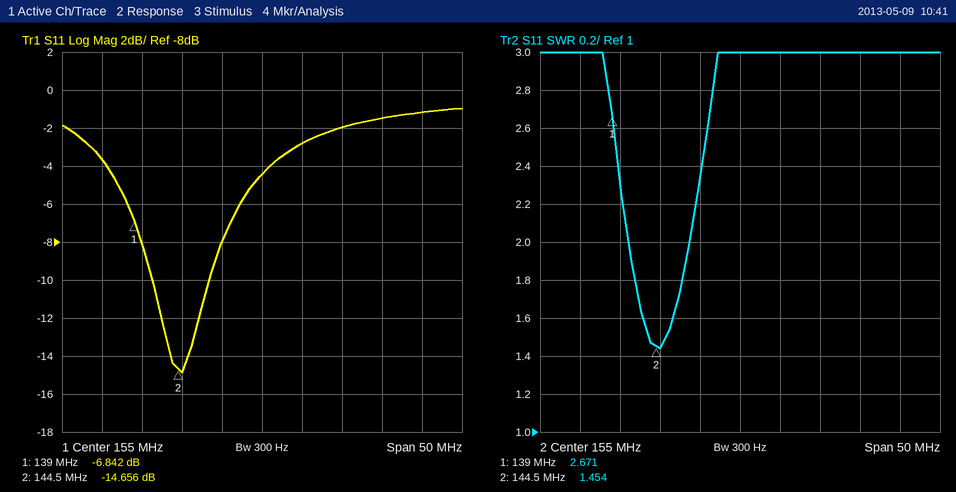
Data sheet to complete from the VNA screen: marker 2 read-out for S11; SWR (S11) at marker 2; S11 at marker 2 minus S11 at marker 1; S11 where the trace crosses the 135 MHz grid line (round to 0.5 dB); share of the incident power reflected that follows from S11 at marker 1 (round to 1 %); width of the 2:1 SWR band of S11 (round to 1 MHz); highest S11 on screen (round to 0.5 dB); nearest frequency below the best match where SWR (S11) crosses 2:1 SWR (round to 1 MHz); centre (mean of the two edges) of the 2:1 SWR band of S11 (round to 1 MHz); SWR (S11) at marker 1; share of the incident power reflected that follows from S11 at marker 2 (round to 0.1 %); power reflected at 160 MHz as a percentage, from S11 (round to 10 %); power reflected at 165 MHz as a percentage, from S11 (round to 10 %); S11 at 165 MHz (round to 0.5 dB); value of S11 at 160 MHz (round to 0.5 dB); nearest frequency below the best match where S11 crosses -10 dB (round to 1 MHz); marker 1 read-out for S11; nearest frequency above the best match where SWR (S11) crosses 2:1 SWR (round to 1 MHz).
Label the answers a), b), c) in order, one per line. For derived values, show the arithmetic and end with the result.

a) -14.656 dB
b) 1.454
c) -14.656 − (-6.842) = -7.814 dB
d) -3.5 dB
e) 10^(-6.842/10) ≈ 21 %
f) 149 MHz − 141 MHz = 8 MHz
g) -1.0 dB
h) 141 MHz
i) 145 MHz
j) 2.671
k) 10^(-14.656/10) ≈ 3.4 %
l) 10^(-3/10) ≈ 50 %
m) 10^(-2/10) ≈ 63.1 %, so 60 % to the nearest 10 %
n) -2.0 dB
o) -3.0 dB
p) 141 MHz
q) -6.842 dB
r) 149 MHz
